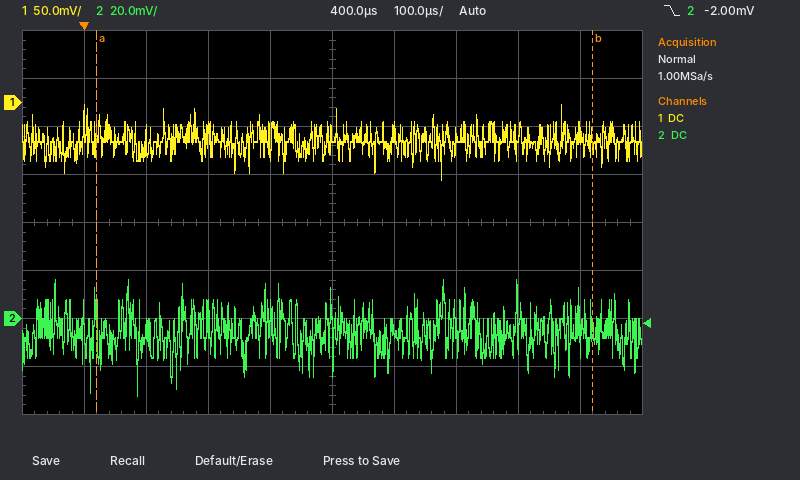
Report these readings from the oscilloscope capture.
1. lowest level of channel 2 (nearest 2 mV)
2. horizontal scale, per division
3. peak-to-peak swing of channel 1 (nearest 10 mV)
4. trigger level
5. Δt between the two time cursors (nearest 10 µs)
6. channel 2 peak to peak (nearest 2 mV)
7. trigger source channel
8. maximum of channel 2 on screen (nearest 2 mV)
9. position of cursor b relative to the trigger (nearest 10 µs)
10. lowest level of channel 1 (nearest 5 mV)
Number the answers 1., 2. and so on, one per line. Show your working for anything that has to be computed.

1. -32 mV
2. 100 µs
3. 80 mV
4. -2.00 mV
5. 800 µs
6. 16 mV − (-32 mV) = 48 mV
7. channel 2
8. 16 mV
9. +820 µs
10. -80 mV
